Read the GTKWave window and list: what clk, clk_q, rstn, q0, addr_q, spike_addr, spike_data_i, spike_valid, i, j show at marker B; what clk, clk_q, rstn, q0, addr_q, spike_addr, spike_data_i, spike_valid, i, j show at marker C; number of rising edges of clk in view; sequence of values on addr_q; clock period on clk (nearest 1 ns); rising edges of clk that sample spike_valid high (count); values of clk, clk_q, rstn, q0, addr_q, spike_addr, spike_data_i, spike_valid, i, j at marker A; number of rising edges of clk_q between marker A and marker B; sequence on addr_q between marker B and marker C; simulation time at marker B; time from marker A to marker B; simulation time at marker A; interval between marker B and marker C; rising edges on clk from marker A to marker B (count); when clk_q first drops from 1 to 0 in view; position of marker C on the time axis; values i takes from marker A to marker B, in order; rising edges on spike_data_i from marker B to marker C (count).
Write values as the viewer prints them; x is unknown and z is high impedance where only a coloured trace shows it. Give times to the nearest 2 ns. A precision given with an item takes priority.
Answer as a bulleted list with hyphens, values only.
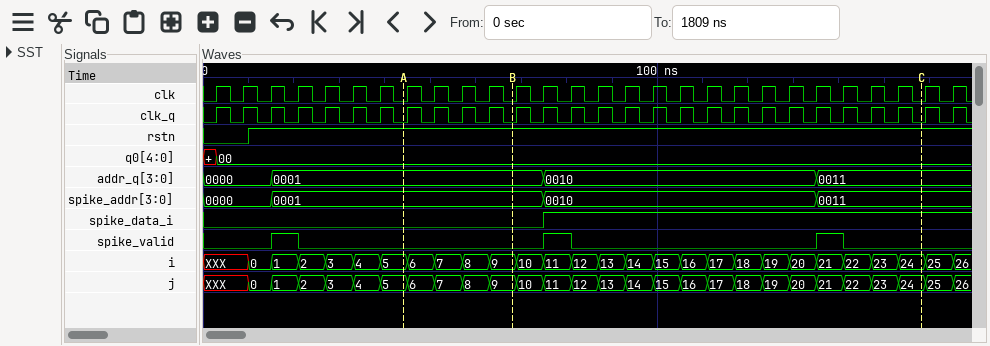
- clk=0, clk_q=0, rstn=1, q0=00, addr_q=0001, spike_addr=0001, spike_data_i=0, spike_valid=0, i=9, j=9
- clk=0, clk_q=0, rstn=1, q0=00, addr_q=0011, spike_addr=0011, spike_data_i=1, spike_valid=0, i=24, j=24
- 28
- 0000, 0001, 0010, 0011
- 6 ns
- 3
- clk=0, clk_q=0, rstn=1, q0=00, addr_q=0001, spike_addr=0001, spike_data_i=0, spike_valid=0, i=5, j=5
- 4
- 0001, 0010, 0011
- 68 ns
- 24 ns
- 44 ns
- 90 ns
- 4
- 6 ns
- 158 ns
- 5, 6, 7, 8, 9
- 1
